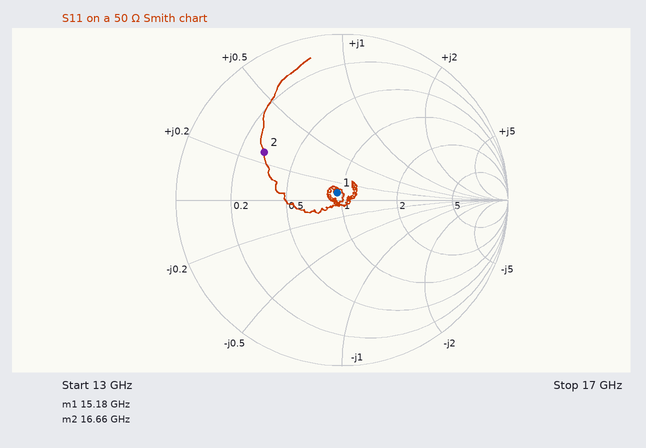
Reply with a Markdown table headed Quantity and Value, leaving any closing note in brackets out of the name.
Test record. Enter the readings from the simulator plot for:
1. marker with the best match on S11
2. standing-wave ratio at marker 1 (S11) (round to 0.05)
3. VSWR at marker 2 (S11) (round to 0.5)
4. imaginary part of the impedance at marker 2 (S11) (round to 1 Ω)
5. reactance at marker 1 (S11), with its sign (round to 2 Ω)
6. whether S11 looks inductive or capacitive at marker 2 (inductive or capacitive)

| Quantity | Value |
|---|---|
| marker with the best match on S11 | marker 1 |
| standing-wave ratio at marker 1 (S11) | 1.10 |
| VSWR at marker 2 (S11) | 3.5 |
| imaginary part of the impedance at marker 2 (S11) | +13 Ω |
| reactance at marker 1 (S11), with its sign | +4 Ω |
| whether S11 looks inductive or capacitive at marker 2 | inductive |
